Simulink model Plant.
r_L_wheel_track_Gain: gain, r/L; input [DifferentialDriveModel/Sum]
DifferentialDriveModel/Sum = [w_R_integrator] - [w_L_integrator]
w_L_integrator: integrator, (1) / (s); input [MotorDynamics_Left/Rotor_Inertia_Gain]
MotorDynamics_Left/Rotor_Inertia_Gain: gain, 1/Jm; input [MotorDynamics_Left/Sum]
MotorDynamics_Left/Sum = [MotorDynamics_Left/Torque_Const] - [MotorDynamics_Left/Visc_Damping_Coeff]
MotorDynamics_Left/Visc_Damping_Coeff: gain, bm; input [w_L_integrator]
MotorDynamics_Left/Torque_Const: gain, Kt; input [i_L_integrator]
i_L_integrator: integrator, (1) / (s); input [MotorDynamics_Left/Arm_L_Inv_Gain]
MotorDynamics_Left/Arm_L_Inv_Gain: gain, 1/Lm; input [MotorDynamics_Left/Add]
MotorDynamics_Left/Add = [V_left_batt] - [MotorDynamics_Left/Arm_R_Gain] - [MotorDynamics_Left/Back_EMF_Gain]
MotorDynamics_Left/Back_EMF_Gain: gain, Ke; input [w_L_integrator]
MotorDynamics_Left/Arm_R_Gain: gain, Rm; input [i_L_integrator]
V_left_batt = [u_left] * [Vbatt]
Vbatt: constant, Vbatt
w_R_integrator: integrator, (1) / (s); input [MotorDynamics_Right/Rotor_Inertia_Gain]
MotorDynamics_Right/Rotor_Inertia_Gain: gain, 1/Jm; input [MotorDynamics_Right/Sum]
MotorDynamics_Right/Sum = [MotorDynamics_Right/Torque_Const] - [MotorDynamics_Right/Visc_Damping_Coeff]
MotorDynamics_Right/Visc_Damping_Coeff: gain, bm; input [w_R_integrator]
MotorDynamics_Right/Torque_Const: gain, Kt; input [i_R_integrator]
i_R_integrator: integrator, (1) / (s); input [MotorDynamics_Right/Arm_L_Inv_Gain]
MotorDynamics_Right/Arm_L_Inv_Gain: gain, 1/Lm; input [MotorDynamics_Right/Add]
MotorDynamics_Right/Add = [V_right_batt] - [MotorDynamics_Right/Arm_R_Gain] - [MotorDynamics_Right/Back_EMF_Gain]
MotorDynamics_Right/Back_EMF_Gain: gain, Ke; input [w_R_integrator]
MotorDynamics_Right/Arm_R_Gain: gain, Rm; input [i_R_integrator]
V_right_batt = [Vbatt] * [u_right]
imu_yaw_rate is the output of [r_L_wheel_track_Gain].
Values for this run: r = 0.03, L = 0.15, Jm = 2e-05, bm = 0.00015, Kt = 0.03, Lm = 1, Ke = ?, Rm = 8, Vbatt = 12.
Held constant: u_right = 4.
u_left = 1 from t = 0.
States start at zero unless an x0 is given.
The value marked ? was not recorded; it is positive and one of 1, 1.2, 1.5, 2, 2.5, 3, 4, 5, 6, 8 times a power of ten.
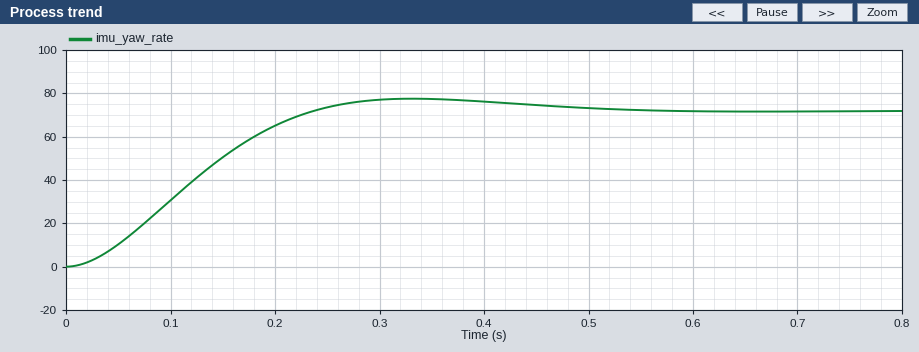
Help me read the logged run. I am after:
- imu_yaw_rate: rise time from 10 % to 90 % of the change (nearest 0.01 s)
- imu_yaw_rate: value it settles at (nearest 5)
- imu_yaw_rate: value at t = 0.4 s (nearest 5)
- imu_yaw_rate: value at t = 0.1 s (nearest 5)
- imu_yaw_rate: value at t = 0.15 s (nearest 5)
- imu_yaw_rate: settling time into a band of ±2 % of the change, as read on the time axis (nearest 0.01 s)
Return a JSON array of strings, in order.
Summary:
["0.16 s", "70", "75", "30", "50", "0.49 s"]
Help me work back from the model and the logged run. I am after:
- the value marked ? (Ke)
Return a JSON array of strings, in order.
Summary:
["0.06"]
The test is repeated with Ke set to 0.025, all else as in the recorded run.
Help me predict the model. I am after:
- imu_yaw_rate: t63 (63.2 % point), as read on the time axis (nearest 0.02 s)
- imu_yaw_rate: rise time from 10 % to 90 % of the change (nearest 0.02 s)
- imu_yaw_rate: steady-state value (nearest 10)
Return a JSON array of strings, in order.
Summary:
["0.18 s", "0.24 s", "110"]
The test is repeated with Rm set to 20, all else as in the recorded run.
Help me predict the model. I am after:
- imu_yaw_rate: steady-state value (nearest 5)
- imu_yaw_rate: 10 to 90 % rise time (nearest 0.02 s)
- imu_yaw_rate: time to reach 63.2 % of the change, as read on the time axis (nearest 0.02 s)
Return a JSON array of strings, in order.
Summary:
["45", "0.18 s", "0.12 s"]
